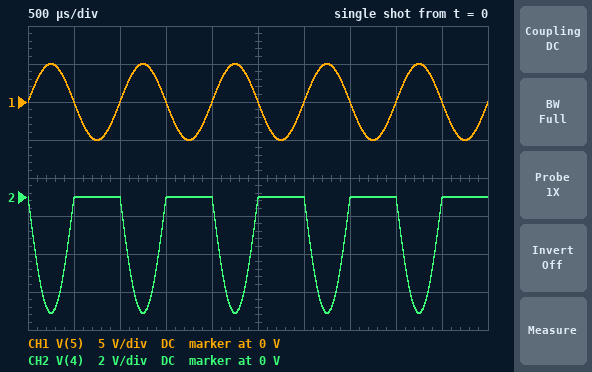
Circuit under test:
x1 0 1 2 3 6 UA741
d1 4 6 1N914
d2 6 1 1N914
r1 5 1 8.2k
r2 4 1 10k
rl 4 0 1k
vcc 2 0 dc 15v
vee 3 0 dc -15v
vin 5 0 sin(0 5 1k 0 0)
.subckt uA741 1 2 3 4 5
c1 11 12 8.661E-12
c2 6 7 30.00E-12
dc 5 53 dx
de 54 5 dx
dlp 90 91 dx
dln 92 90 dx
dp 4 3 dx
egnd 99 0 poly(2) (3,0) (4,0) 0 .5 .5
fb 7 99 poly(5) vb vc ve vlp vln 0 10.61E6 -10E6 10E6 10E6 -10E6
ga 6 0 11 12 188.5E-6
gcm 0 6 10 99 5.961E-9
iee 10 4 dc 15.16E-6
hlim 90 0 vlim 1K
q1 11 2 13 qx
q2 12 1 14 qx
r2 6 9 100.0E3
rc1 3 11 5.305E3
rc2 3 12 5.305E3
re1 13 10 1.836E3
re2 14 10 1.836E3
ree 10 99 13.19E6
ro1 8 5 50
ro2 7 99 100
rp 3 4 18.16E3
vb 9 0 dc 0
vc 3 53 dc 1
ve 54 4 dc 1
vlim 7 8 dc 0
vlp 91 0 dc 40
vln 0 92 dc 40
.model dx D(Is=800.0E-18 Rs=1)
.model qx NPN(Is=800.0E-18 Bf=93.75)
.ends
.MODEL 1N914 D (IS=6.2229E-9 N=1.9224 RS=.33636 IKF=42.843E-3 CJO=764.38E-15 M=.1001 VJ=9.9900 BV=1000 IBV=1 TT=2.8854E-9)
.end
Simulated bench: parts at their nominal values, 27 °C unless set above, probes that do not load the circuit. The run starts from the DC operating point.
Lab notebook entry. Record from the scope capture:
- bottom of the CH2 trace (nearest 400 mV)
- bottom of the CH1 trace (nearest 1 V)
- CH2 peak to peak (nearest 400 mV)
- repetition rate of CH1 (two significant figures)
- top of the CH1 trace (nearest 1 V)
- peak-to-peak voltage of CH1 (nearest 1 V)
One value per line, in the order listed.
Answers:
-6.0 V
-5 V
6.0 V
1.0 kHz
5 V
10 V
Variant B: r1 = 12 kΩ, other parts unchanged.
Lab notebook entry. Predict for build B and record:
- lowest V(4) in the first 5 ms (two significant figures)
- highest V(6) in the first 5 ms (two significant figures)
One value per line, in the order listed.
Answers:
-4.2 V
560 mV
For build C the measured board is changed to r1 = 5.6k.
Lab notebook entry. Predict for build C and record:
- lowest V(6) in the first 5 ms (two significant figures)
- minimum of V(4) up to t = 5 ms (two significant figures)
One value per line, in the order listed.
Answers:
-9.7 V
-8.9 V
